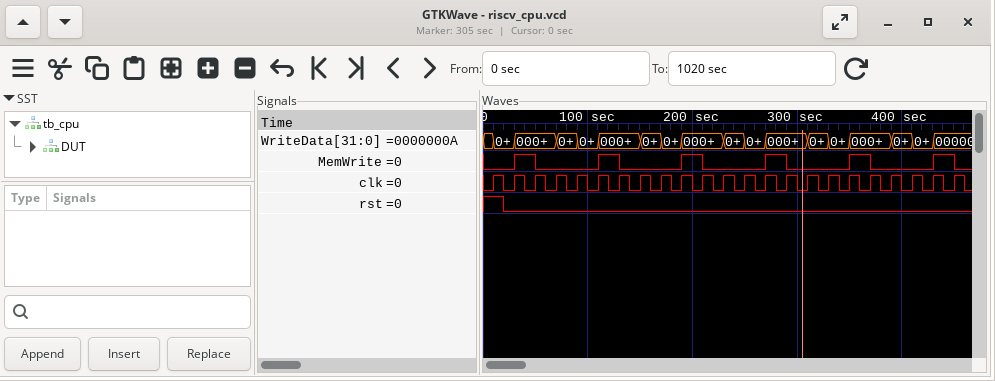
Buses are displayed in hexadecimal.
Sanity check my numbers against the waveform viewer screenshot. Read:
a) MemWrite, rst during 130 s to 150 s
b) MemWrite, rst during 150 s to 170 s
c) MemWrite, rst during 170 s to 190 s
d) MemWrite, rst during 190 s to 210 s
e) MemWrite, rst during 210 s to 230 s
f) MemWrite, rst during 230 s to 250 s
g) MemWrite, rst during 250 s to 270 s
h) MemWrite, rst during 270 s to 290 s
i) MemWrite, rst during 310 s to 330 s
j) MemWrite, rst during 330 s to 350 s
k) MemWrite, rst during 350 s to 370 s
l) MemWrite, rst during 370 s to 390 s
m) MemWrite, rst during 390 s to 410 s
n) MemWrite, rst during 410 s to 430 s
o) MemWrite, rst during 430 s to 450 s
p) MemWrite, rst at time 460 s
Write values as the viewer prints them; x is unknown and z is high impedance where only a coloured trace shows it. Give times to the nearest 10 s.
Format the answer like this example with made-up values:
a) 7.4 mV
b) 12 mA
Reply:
a) MemWrite=0, rst=0
b) MemWrite=0, rst=0
c) MemWrite=0, rst=0
d) MemWrite=1, rst=0
e) MemWrite=0, rst=0
f) MemWrite=0, rst=0
g) MemWrite=0, rst=0
h) MemWrite=1, rst=0
i) MemWrite=0, rst=0
j) MemWrite=0, rst=0
k) MemWrite=1, rst=0
l) MemWrite=0, rst=0
m) MemWrite=0, rst=0
n) MemWrite=0, rst=0
o) MemWrite=1, rst=0
p) MemWrite=0, rst=0
